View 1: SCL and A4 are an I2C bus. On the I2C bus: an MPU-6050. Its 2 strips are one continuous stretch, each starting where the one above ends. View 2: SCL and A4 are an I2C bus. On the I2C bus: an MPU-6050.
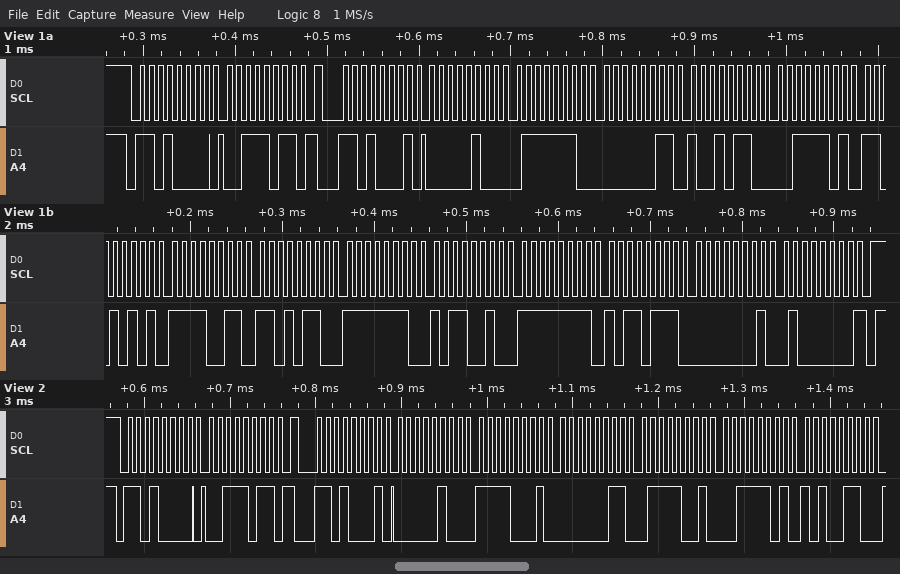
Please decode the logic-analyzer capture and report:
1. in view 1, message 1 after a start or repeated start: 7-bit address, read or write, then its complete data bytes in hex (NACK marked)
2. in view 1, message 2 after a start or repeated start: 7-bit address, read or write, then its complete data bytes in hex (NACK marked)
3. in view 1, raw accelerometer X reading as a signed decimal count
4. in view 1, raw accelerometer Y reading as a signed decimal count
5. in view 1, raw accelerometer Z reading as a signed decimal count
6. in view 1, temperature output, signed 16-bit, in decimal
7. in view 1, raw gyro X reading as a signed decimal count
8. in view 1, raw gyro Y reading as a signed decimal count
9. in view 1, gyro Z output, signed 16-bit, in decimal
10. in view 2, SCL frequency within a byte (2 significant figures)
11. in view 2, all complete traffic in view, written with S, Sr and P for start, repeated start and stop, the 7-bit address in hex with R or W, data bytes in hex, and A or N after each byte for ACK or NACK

0x68 write: 3B
0x68 read: 04 7E 03 96 3D D5 F3 D6 FE B2 FF B7 01 40 NACK
1150
918
15829
-3114
-334
-73
320
100 kHz
S 68W A 3B A Sr 68R A 04 A F1 A 03 A 79 A 3D A A6 A
